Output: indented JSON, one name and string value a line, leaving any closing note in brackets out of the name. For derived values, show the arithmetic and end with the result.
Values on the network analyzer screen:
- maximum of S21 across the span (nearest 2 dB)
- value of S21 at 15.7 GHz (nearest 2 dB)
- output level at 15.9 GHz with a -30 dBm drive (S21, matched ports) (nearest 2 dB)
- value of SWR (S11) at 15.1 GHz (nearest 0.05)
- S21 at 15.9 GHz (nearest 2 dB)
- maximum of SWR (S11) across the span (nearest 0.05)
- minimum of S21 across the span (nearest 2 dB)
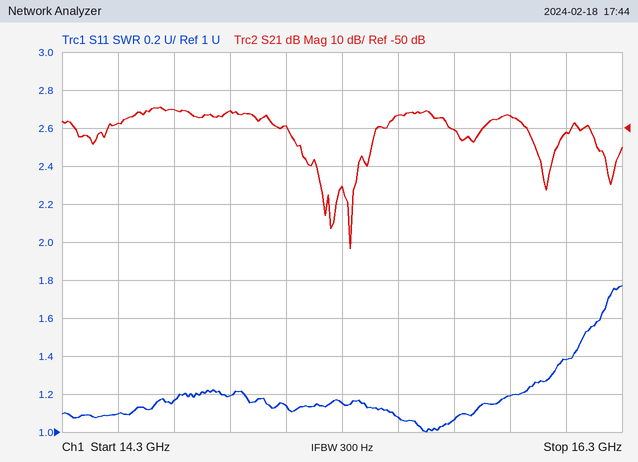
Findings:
{
  "maximum of S21 across the span": "-44 dB",
  "value of S21 at 15.7 GHz": "-50 dB",
  "output level at 15.9 GHz with a -30 dBm drive (S21, matched ports)": "-30 dBm + (-46 dB) = -76 dBm",
  "value of SWR (S11) at 15.1 GHz": "1.15",
  "S21 at 15.9 GHz": "-46 dB",
  "maximum of SWR (S11) across the span": "1.75",
  "minimum of S21 across the span": "-82 dB"
}
